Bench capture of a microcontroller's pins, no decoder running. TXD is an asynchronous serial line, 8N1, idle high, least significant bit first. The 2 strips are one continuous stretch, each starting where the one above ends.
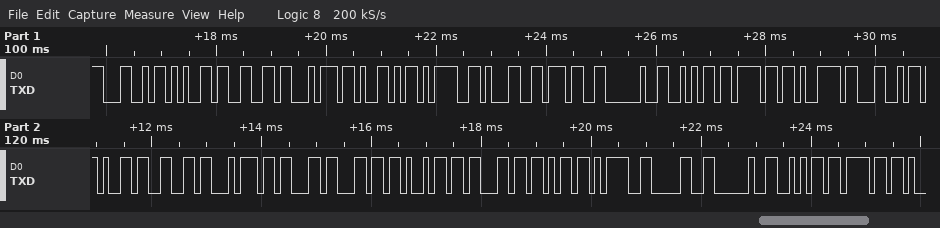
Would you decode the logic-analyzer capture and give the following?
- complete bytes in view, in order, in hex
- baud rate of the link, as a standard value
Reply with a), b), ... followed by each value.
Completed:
a) 4C 65 66 74 59 3D 31 37 20 6A 6F 79 4C 65 66 74 63 6C 69 63 6B 3D 30 20 6A 6F
b) 9600 baud
